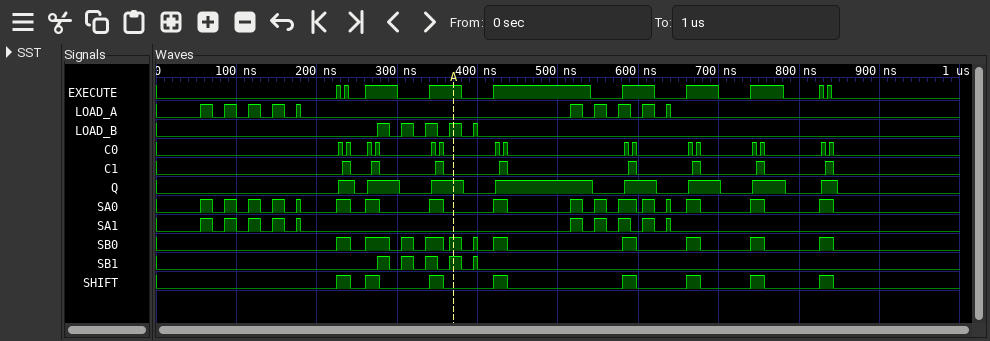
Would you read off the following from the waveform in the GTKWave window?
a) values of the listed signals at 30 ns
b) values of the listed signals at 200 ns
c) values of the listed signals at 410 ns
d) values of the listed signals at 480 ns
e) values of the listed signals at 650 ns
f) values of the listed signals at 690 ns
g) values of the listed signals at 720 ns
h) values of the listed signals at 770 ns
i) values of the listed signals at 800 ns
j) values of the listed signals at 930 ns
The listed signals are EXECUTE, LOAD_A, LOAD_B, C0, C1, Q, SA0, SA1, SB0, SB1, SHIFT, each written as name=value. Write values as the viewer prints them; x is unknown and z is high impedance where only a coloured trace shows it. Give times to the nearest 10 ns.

EXECUTE=0, LOAD_A=0, LOAD_B=0, C0=0, C1=0, Q=0, SA0=0, SA1=0, SB0=0, SB1=0, SHIFT=0
EXECUTE=0, LOAD_A=0, LOAD_B=0, C0=0, C1=0, Q=0, SA0=0, SA1=0, SB0=0, SB1=0, SHIFT=0
EXECUTE=0, LOAD_A=0, LOAD_B=0, C0=0, C1=0, Q=0, SA0=0, SA1=0, SB0=0, SB1=0, SHIFT=0
EXECUTE=1, LOAD_A=0, LOAD_B=0, C0=0, C1=0, Q=1, SA0=0, SA1=0, SB0=0, SB1=0, SHIFT=0
EXECUTE=0, LOAD_A=0, LOAD_B=0, C0=0, C1=0, Q=0, SA0=0, SA1=0, SB0=0, SB1=0, SHIFT=0
EXECUTE=1, LOAD_A=0, LOAD_B=0, C0=0, C1=0, Q=1, SA0=0, SA1=0, SB0=0, SB1=0, SHIFT=0
EXECUTE=0, LOAD_A=0, LOAD_B=0, C0=0, C1=0, Q=0, SA0=0, SA1=0, SB0=0, SB1=0, SHIFT=0
EXECUTE=1, LOAD_A=0, LOAD_B=0, C0=0, C1=0, Q=1, SA0=0, SA1=0, SB0=0, SB1=0, SHIFT=0
EXECUTE=0, LOAD_A=0, LOAD_B=0, C0=0, C1=0, Q=0, SA0=0, SA1=0, SB0=0, SB1=0, SHIFT=0
EXECUTE=0, LOAD_A=0, LOAD_B=0, C0=0, C1=0, Q=0, SA0=0, SA1=0, SB0=0, SB1=0, SHIFT=0
